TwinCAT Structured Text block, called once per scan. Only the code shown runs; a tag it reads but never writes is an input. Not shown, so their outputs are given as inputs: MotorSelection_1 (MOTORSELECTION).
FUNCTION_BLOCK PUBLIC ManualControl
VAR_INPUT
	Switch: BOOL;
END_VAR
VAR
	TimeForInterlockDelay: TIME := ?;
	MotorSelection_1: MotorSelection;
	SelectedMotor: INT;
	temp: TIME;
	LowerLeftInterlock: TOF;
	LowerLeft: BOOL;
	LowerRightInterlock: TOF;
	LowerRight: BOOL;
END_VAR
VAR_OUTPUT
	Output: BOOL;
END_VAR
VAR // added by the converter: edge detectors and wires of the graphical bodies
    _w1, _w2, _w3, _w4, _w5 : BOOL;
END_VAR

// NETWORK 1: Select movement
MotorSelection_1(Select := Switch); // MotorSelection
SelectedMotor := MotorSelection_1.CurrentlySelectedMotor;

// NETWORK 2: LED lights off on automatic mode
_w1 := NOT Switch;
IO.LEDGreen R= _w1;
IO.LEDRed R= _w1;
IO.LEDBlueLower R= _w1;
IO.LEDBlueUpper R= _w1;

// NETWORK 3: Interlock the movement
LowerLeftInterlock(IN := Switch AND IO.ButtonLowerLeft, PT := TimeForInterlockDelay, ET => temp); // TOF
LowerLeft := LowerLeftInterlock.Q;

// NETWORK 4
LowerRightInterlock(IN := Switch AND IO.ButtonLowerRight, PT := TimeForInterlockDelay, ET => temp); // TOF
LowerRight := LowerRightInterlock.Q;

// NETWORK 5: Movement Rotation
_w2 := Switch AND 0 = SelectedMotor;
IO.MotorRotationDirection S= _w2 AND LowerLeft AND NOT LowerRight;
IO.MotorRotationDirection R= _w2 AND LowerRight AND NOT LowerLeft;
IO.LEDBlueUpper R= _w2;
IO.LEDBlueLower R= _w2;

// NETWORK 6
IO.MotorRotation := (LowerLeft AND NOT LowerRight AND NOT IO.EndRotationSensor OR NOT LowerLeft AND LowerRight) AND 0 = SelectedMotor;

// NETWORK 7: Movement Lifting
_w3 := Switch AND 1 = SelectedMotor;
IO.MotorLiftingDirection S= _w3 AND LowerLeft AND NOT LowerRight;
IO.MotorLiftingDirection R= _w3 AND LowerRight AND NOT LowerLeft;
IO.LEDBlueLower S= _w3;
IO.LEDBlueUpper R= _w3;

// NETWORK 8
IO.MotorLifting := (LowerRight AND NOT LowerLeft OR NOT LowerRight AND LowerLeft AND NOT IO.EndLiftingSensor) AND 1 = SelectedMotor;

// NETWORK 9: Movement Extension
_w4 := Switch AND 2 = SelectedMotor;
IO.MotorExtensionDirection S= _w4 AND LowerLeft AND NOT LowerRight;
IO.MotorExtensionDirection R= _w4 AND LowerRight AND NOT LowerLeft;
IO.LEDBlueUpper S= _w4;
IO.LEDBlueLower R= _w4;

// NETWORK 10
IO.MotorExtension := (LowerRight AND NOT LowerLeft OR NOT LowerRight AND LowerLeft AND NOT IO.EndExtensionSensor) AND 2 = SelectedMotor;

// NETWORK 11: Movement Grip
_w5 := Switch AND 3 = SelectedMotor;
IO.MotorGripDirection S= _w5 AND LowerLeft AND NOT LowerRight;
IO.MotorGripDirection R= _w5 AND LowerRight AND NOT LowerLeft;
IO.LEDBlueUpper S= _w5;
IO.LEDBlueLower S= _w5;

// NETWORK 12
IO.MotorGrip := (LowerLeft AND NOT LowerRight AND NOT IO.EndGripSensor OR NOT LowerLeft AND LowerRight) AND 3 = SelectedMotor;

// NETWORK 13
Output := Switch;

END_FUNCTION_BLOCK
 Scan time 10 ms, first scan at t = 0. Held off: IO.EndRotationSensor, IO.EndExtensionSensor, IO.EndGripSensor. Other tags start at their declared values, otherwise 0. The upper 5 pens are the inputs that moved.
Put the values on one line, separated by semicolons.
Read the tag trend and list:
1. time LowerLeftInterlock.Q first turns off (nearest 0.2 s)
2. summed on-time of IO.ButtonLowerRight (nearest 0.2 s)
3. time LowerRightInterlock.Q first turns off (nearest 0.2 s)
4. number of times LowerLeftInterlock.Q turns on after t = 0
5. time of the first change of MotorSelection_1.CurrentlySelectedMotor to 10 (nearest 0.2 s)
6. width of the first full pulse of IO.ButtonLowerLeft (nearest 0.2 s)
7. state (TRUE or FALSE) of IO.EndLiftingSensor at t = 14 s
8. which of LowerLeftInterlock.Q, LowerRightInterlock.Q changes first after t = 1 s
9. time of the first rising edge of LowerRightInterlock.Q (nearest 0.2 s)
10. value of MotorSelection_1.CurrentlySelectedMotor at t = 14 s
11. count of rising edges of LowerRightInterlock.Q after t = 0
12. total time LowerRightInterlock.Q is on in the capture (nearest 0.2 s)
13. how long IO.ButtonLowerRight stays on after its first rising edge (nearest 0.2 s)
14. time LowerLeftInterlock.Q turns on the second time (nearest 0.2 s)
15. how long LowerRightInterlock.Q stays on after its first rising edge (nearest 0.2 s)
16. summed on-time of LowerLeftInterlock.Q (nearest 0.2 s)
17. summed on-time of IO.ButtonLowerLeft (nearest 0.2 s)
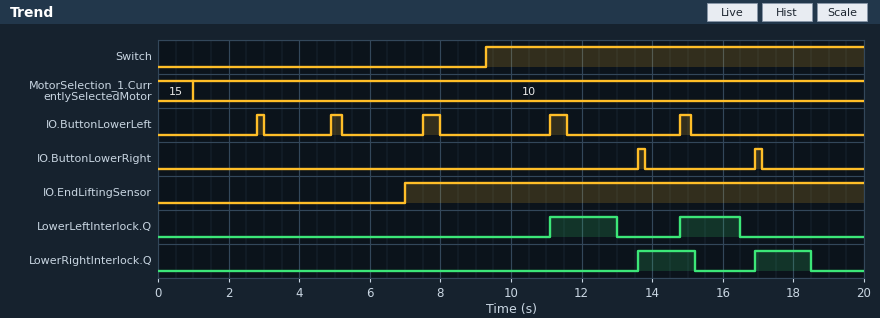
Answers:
13.0 s; 0.4 s; 15.2 s; 2; 1.0 s; 0.2 s; TRUE; LowerLeftInterlock.Q; 13.6 s; 10; 2; 3.2 s; 0.2 s; 14.8 s; 1.6 s; 3.6 s; 1.8 s
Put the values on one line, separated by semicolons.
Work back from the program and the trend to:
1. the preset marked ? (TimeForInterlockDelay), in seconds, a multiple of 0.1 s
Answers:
1.4 s
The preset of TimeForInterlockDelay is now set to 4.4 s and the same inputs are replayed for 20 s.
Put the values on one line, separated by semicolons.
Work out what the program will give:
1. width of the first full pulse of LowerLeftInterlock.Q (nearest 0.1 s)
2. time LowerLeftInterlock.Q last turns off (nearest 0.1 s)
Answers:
8.4 s; 19.5 s
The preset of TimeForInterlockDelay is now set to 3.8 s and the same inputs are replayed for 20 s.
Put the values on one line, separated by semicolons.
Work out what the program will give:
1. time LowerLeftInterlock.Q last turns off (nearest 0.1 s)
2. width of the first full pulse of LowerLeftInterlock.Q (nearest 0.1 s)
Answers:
18.9 s; 7.8 s
